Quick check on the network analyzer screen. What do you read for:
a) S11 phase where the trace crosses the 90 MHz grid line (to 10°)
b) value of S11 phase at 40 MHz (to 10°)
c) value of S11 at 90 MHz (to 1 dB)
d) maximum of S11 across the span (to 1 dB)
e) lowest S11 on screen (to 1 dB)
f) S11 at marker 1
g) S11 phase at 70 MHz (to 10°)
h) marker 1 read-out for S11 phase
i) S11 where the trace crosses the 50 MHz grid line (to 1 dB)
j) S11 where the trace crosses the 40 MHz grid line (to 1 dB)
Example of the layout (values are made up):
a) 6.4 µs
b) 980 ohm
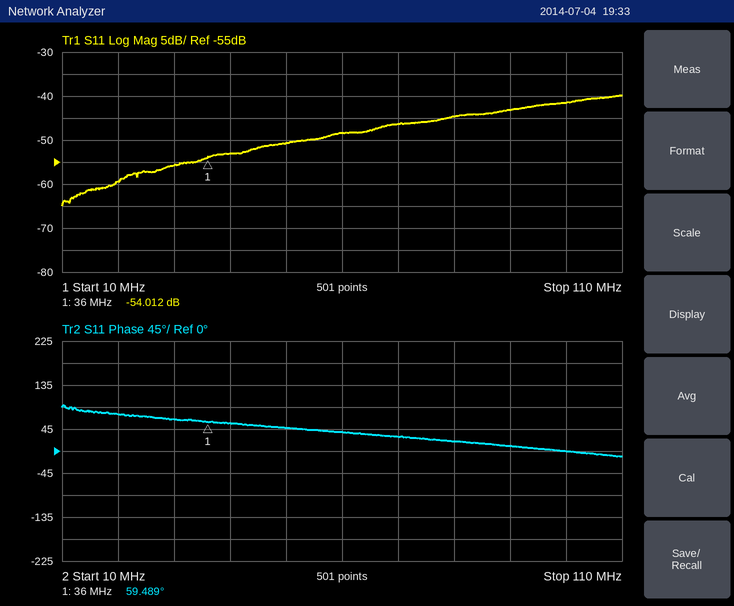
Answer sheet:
a) 10°
b) 60°
c) -43 dB
d) -40 dB
e) -65 dB
f) -54.012 dB
g) 30°
h) 59.489°
i) -51 dB
j) -53 dB
